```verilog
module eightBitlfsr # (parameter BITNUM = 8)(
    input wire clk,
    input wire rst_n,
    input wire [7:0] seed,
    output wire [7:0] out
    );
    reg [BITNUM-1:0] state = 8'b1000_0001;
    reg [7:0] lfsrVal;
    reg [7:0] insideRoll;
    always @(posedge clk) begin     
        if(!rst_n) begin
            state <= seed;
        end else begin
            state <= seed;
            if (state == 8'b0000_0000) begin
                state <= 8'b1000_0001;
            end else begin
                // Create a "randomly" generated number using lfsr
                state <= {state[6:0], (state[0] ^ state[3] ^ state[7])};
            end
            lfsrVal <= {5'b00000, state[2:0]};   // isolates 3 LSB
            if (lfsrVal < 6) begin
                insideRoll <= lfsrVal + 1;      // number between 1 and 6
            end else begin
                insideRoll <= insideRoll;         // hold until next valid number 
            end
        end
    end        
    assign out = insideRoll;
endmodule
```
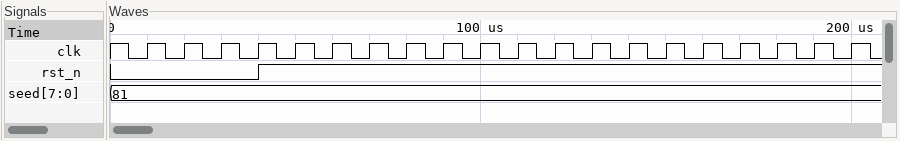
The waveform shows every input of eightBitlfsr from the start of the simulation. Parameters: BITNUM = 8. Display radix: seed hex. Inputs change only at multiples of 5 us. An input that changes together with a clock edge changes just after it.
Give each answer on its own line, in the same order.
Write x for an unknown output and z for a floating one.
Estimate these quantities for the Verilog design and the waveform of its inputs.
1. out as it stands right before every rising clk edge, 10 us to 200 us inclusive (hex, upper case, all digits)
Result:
x, x, x, x, x, x, 02, 03, 05, 01, 02, 04, 04, 04, 04, 04, 06, 03, 05, 02
